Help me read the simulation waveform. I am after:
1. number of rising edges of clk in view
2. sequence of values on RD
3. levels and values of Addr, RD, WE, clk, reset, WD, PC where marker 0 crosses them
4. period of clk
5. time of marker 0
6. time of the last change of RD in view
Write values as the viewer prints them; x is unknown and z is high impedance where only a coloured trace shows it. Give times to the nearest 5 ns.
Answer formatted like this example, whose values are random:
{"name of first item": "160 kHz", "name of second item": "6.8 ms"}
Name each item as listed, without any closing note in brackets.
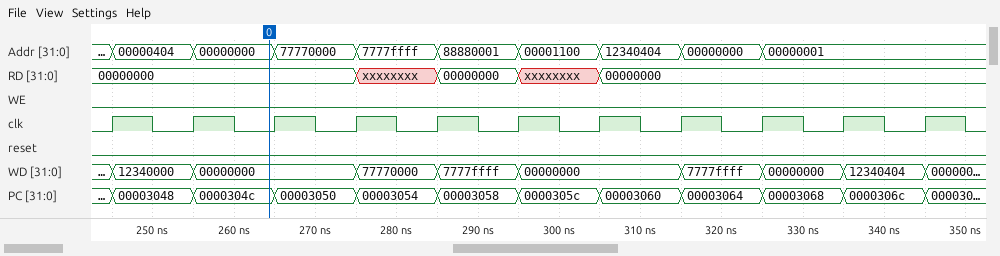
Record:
{"number of rising edges of clk in view": "11", "sequence of values on RD": "00000000, xxxxxxxx, 00000000, xxxxxxxx, 00000000", "levels and values of Addr, RD, WE, clk, reset, WD, PC where marker 0 crosses them": "Addr=00000000, RD=00000000, WE=0, clk=0, reset=0, WD=00000000, PC=0000304c", "period of clk": "10 ns", "time of marker 0": "265 ns", "time of the last change of RD in view": "305 ns"}
